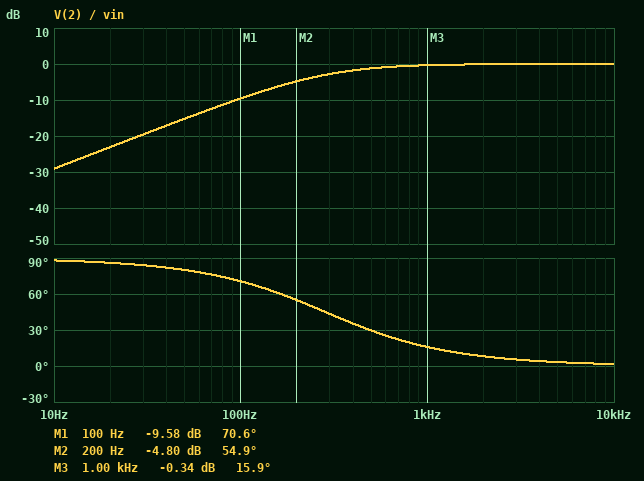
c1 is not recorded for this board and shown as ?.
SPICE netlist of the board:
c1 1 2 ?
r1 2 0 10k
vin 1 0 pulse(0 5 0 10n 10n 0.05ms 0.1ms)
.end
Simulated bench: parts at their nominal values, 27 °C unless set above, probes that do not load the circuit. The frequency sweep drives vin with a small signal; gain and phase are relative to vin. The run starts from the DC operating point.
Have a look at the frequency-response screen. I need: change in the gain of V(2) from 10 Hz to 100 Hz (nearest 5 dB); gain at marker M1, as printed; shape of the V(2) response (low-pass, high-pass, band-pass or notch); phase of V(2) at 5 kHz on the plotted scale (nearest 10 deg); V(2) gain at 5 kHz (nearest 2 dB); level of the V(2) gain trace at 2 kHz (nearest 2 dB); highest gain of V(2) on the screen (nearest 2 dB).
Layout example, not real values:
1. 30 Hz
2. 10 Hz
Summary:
1. 20 dB
2. -9.58 dB
3. high-pass
4. 0 deg
5. 0 dB
6. 0 dB
7. 0 dB
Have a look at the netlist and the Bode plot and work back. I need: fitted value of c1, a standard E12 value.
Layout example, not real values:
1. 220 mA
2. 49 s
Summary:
1. 56 nF
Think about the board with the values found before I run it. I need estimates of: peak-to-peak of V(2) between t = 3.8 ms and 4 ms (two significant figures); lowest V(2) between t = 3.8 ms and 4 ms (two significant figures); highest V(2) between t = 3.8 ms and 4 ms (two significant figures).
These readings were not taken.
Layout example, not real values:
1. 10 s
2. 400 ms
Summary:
1. 5.2 V
2. -2.6 V
3. 2.6 V
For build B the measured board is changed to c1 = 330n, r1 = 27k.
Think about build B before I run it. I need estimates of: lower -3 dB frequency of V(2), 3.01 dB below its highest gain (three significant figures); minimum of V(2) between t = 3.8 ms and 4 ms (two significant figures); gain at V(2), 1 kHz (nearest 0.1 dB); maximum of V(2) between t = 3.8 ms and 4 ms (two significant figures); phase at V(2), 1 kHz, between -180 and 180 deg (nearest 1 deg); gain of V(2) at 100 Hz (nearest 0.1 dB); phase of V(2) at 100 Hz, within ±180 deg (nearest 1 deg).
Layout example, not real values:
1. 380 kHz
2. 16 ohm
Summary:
1. 17.9 Hz
2. -910 mV
3. 0 dB
4. 4.1 V
5. 1 deg
6. -0.1 dB
7. 10 deg
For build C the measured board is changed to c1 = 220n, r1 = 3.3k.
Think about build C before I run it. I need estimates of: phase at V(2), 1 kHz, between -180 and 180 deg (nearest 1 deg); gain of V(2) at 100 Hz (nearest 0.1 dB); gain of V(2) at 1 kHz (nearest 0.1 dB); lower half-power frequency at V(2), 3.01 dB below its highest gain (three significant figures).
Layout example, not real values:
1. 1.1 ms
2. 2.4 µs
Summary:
1. 12 deg
2. -7.6 dB
3. -0.2 dB
4. 219 Hz
